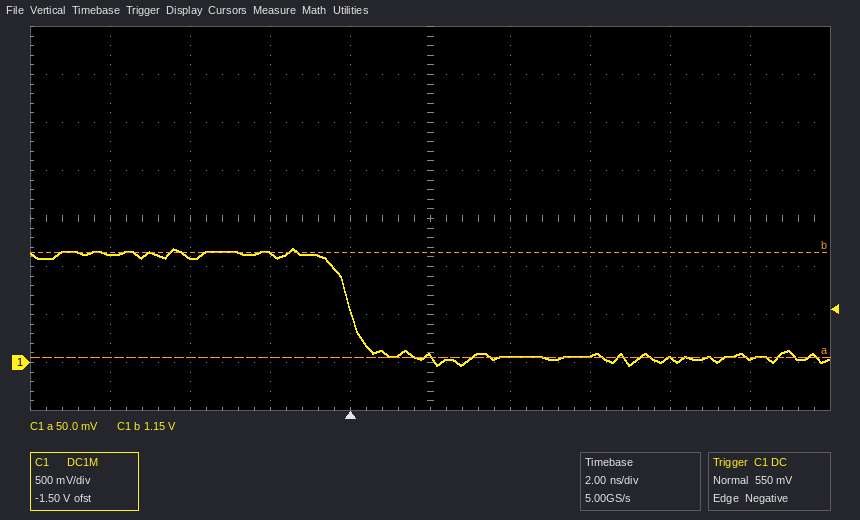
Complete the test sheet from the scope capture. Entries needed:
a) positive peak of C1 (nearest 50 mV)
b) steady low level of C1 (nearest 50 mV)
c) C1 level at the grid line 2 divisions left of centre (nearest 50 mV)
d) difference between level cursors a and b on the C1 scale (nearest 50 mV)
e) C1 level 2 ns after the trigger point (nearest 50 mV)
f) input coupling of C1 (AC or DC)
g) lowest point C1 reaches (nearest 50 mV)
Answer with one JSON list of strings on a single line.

["1.20 V", "50 mV", "1.15 V", "1.10 V", "50 mV", "DC", "-50 mV"]
